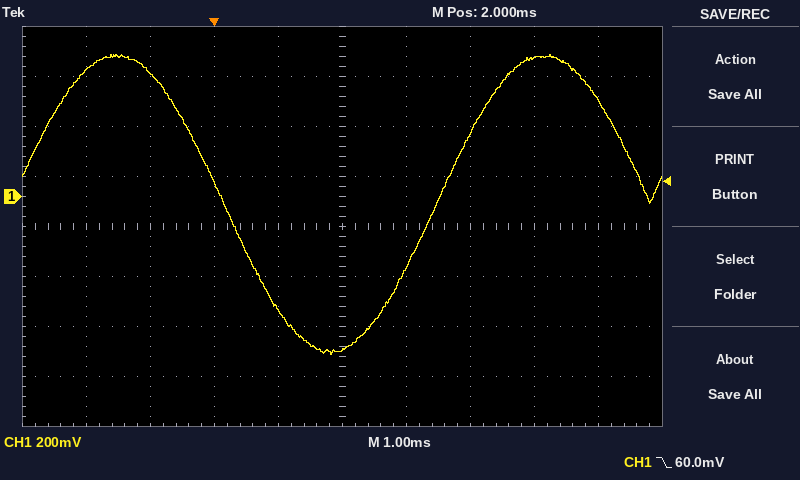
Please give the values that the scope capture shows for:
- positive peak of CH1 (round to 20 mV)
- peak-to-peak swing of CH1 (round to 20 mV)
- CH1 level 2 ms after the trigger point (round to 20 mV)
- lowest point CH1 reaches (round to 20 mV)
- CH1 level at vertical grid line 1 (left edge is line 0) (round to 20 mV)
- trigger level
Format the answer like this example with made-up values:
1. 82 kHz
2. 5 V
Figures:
1. 560 mV
2. 1.20 V
3. -620 mV
4. -640 mV
5. 500 mV
6. 60.0 mV
